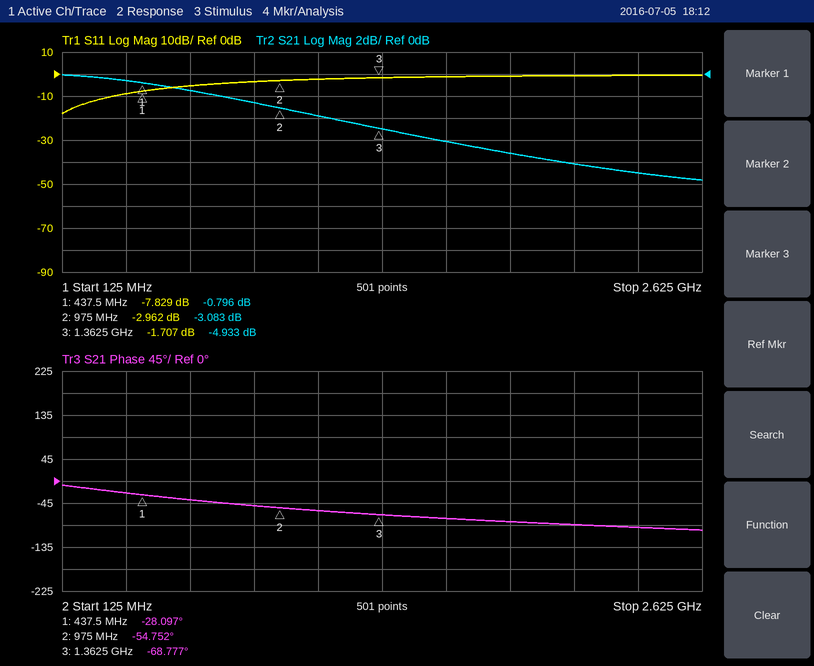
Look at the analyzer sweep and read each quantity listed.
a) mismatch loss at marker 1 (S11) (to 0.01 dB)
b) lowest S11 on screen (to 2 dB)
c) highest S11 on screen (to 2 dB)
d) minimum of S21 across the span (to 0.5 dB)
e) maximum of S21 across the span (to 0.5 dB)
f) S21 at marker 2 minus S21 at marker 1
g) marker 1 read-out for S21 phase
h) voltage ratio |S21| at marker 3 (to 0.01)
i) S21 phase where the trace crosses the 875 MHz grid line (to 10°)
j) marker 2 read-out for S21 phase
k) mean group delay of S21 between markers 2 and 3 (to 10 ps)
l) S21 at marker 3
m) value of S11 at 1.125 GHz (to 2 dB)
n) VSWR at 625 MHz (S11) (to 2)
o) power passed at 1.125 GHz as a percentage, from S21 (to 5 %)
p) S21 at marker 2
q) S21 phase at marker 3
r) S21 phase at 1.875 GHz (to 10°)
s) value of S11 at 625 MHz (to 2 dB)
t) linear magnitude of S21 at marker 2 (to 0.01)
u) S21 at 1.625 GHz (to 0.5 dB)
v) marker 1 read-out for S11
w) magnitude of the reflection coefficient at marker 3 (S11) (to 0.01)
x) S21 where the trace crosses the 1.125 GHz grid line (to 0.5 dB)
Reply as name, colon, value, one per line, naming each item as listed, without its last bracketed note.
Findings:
mismatch loss at marker 1 (S11): 0.78 dB
lowest S11 on screen: -18 dB
highest S11 on screen: 0 dB
minimum of S21 across the span: -9.5 dB
maximum of S21 across the span: 0.0 dB
S21 at marker 2 minus S21 at marker 1: -2.287 dB
marker 1 read-out for S21 phase: -28.097°
voltage ratio |S21| at marker 3: 0.57
S21 phase where the trace crosses the 875 MHz grid line: -50°
marker 2 read-out for S21 phase: -54.752°
mean group delay of S21 between markers 2 and 3: 100 ps
S21 at marker 3: -4.933 dB
value of S11 at 1.125 GHz: -2 dB
VSWR at 625 MHz (S11): 4
power passed at 1.125 GHz as a percentage, from S21: 40 %
S21 at marker 2: -3.083 dB
S21 phase at marker 3: -68.777°
S21 phase at 1.875 GHz: -80°
value of S11 at 625 MHz: -6 dB
linear magnitude of S21 at marker 2: 0.70
S21 at 1.625 GHz: -6.0 dB
marker 1 read-out for S11: -7.829 dB
magnitude of the reflection coefficient at marker 3 (S11): 0.82
S21 where the trace crosses the 1.125 GHz grid line: -4.0 dB
